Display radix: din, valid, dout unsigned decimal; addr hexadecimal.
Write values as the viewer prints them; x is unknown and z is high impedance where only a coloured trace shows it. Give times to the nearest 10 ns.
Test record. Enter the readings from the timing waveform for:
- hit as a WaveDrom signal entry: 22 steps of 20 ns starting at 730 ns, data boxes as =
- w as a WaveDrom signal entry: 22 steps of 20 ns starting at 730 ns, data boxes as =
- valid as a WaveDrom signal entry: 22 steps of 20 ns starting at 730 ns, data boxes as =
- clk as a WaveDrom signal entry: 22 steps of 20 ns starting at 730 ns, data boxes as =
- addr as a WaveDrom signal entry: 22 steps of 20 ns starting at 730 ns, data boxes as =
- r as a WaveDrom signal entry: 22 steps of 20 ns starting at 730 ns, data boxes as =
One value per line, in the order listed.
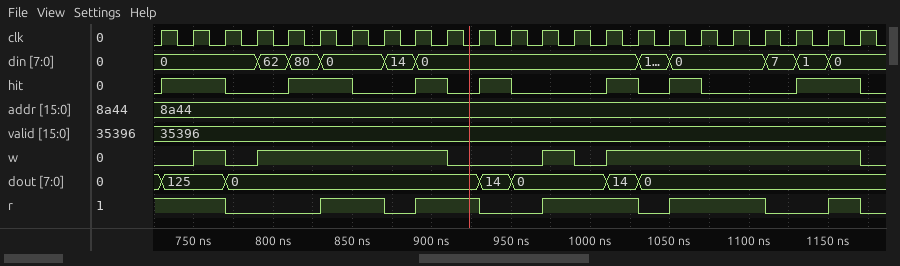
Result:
{name: 'hit', wave: '1.0.1.0.1010..1010..1.'}
{name: 'w', wave: '0101.....0..101.......'}
{name: 'valid', wave: '=.....................', data: '35396'}
{name: 'clk', wave: 'p.....................'}
{name: 'addr', wave: '=.....................', data: '8a44'}
{name: 'r', wave: '1.0..1.01.0.1..01..0.1'}
